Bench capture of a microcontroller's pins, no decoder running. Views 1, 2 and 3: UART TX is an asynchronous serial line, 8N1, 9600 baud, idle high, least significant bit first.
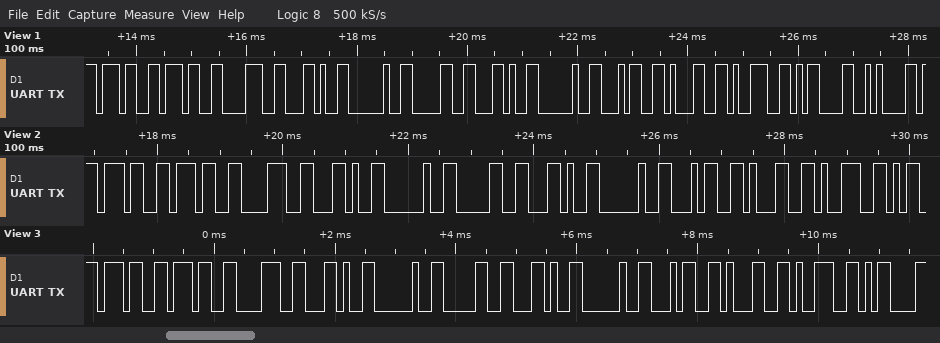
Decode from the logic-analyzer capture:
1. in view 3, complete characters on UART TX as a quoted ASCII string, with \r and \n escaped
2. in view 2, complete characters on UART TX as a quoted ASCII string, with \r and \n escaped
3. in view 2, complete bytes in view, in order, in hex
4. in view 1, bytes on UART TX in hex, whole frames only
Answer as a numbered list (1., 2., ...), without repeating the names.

1. "778, 0, 419\r"
2. "778, 0, 419"
3. 0x37 0x37 0x38 0x2C 0x20 0x30 0x2C 0x20 0x34 0x31 0x39
4. 0x37 0x37 0x38 0x2C 0x20 0x30 0x2C 0x20 0x34 0x31 0x39 0x0D 0x0A
